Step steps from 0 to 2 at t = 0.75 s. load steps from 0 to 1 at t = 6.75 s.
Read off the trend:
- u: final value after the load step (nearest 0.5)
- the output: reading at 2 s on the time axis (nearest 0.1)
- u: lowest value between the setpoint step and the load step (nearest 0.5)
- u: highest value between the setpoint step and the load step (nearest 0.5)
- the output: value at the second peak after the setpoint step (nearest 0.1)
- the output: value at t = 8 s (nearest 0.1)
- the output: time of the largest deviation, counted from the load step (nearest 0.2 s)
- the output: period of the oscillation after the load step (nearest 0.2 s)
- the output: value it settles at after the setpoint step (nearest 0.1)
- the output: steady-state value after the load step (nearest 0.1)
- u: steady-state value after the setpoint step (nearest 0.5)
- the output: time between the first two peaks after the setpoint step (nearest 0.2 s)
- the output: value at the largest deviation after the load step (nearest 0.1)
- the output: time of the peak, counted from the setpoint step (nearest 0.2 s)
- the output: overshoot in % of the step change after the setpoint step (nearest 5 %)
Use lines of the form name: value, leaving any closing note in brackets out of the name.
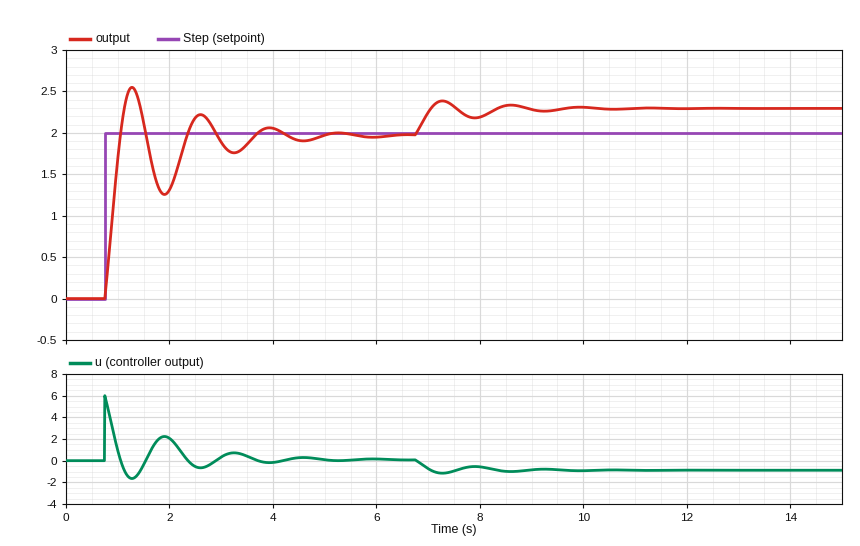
u: final value after the load step: -1.0
the output: reading at 2 s on the time axis: 1.3
u: lowest value between the setpoint step and the load step: -1.5
u: highest value between the setpoint step and the load step: 6.0
the output: value at the second peak after the setpoint step: 2.2
the output: value at t = 8 s: 2.2
the output: time of the largest deviation, counted from the load step: 0.6 s
the output: period of the oscillation after the load step: 1.4 s
the output: value it settles at after the setpoint step: 2.0
the output: steady-state value after the load step: 2.3
u: steady-state value after the setpoint step: 0.0
the output: time between the first two peaks after the setpoint step: 1.4 s
the output: value at the largest deviation after the load step: 2.4
the output: time of the peak, counted from the setpoint step: 0.6 s
the output: overshoot in % of the step change after the setpoint step: 30 %
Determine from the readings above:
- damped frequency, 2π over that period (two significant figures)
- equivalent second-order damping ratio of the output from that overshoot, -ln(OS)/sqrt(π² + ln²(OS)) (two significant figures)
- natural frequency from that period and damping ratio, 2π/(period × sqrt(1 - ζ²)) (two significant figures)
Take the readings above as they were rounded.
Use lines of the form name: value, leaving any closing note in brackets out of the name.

damped frequency, 2π over that period: 4.5 rad/s
equivalent second-order damping ratio of the output from that overshoot, -ln(OS)/sqrt(π² + ln²(OS)): 0.36
natural frequency from that period and damping ratio, 2π/(period × sqrt(1 - ζ²)): 4.8 rad/s
